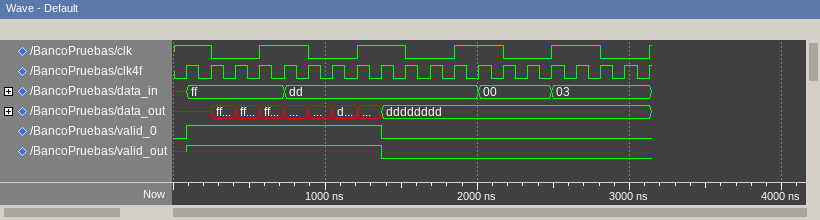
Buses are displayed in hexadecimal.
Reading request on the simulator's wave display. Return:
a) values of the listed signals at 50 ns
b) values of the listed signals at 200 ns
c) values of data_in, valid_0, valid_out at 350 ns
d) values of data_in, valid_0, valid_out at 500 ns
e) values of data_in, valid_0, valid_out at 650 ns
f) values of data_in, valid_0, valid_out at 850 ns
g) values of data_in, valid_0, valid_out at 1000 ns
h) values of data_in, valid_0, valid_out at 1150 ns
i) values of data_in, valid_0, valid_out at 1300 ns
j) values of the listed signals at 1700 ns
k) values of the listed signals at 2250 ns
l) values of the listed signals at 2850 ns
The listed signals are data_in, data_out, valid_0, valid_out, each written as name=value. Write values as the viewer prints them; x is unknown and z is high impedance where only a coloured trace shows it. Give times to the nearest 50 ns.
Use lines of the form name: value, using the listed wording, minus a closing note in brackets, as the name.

values of the listed signals at 50 ns: data_in=x, data_out=x, valid_0=0, valid_out=x
values of the listed signals at 200 ns: data_in=ff, data_out=x, valid_0=1, valid_out=1
values of data_in, valid_0, valid_out at 350 ns: data_in=ff, valid_0=1, valid_out=1
values of data_in, valid_0, valid_out at 500 ns: data_in=ff, valid_0=1, valid_out=1
values of data_in, valid_0, valid_out at 650 ns: data_in=ff, valid_0=1, valid_out=1
values of data_in, valid_0, valid_out at 850 ns: data_in=dd, valid_0=1, valid_out=1
values of data_in, valid_0, valid_out at 1000 ns: data_in=dd, valid_0=1, valid_out=1
values of data_in, valid_0, valid_out at 1150 ns: data_in=dd, valid_0=1, valid_out=1
values of data_in, valid_0, valid_out at 1300 ns: data_in=dd, valid_0=1, valid_out=1
values of the listed signals at 1700 ns: data_in=dd, data_out=dddddddd, valid_0=0, valid_out=0
values of the listed signals at 2250 ns: data_in=00, data_out=dddddddd, valid_0=0, valid_out=0
values of the listed signals at 2850 ns: data_in=03, data_out=dddddddd, valid_0=0, valid_out=0
